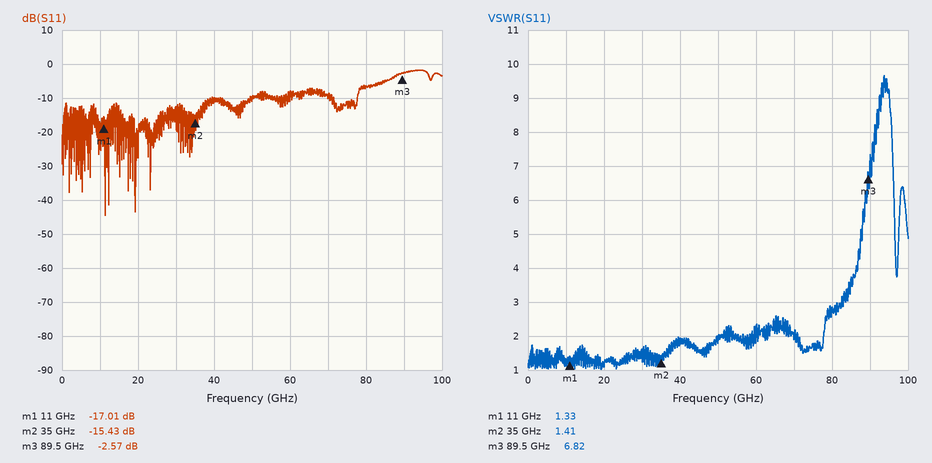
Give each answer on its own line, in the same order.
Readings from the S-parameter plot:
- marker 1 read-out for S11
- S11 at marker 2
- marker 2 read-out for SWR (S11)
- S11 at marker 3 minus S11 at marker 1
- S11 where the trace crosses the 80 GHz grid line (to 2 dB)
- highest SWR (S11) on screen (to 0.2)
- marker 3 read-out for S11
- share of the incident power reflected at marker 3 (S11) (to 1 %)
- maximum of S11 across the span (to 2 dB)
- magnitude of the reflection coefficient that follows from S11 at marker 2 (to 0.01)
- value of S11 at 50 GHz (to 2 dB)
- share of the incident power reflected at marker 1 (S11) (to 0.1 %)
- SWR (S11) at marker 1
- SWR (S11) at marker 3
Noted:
-17.01 dB
-15.43 dB
1.41
14.44 dB
-6 dB
9.6
-2.57 dB
55 %
-2 dB
0.17
-10 dB
2.0 %
1.33
6.82
